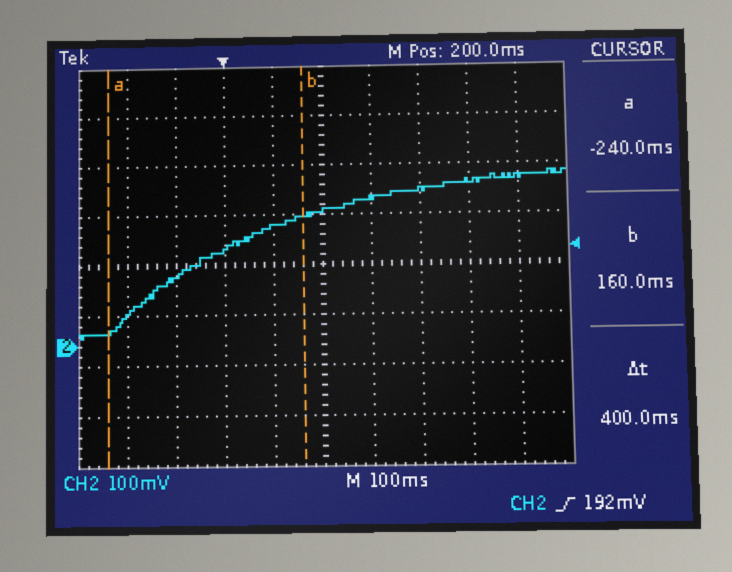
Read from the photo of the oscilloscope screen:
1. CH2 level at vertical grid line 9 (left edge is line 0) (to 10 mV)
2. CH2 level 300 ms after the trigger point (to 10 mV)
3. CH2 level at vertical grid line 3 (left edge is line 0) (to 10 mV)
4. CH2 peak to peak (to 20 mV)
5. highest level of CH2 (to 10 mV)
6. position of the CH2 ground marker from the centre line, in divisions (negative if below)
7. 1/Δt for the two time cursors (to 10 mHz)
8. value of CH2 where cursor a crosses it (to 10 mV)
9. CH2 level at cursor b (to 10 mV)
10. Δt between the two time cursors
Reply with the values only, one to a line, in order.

330 mV
290 mV
190 mV
320 mV
340 mV
-1.6 div
2.50 Hz
30 mV
260 mV
400 ms
